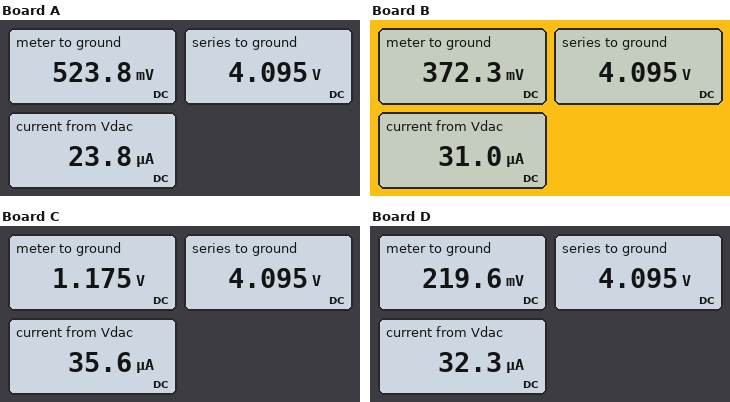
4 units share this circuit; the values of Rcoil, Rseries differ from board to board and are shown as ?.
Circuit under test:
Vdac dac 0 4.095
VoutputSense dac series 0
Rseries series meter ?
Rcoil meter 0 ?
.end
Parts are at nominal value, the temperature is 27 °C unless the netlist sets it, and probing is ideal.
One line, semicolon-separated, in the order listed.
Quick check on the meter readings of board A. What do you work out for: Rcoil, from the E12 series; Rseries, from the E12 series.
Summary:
22 kΩ; 150 kΩ
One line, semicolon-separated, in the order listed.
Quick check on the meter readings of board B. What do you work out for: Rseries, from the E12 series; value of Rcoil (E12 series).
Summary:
120 kΩ; 12 kΩ
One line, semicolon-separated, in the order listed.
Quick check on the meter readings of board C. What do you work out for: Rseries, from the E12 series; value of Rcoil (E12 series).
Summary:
82 kΩ; 33 kΩ
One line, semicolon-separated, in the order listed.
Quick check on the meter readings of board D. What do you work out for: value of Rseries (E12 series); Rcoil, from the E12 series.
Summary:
120 kΩ; 6.8 kΩ
